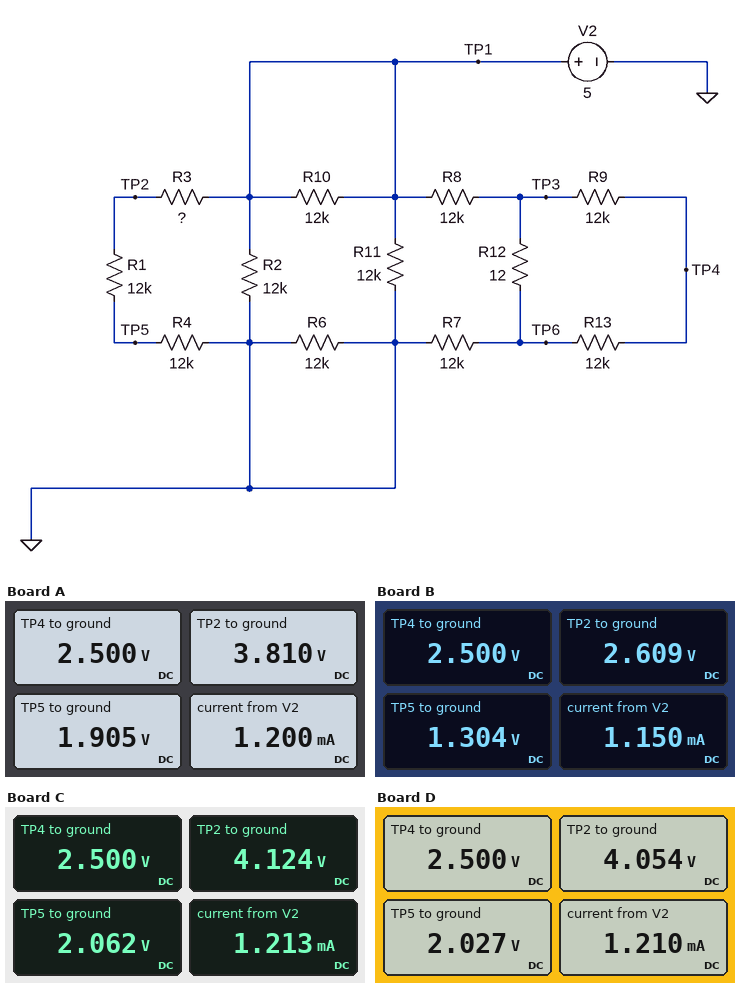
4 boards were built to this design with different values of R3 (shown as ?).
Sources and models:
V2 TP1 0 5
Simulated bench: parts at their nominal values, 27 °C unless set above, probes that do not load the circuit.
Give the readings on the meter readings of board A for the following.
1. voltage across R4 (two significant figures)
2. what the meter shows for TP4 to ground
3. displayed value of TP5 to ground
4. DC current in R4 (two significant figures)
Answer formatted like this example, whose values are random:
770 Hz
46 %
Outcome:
1.9 V
2.500 V
1.905 V
160 µA
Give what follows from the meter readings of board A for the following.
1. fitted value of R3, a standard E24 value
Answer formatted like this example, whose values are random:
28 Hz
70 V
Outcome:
7.5 kΩ
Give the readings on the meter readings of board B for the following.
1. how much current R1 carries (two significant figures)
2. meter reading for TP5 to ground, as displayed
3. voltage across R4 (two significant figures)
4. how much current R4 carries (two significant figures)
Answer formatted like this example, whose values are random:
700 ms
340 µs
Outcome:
110 µA
1.304 V
1.3 V
110 µA
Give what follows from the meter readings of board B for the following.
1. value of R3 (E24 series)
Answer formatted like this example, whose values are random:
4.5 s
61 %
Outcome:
22 kΩ
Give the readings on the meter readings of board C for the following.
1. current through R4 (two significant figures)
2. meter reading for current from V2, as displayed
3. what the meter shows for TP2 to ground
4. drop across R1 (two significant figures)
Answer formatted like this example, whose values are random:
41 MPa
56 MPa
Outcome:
170 µA
1.213 mA
4.124 V
2.1 V
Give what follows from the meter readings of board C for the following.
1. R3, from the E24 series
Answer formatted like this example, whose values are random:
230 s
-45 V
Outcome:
5.1 kΩ
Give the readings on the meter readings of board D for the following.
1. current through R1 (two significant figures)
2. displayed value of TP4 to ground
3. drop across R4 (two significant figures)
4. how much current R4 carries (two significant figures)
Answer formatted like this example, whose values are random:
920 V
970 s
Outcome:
170 µA
2.500 V
2.0 V
170 µA
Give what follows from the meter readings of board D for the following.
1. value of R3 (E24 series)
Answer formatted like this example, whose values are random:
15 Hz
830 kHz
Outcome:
5.6 kΩ
